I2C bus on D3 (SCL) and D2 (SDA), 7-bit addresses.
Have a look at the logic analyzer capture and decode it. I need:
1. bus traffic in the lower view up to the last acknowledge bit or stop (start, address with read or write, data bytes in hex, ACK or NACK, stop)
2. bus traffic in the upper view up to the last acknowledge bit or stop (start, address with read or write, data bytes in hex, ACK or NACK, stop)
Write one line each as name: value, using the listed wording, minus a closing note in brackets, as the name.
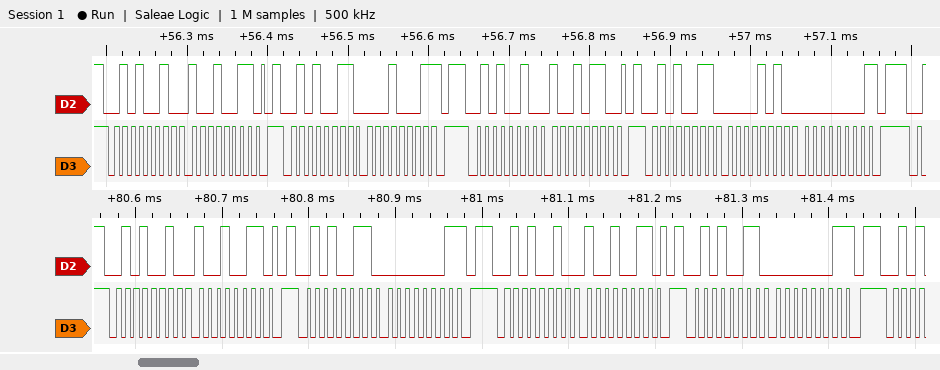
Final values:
bus traffic in the lower view up to the last acknowledge bit or stop: start, address 29 write ACK, 93 ACK, stop, start, address 29 read ACK, 01 NACK, stop, start, address 29 write ACK, 93 ACK, stop, start, address 29 read ACK, 01 NACK, stop
bus traffic in the upper view up to the last acknowledge bit or stop: start, address 29 write ACK, 93 ACK, stop, start, address 29 read ACK, 11 NACK, stop, start, address 29 write ACK, 96 ACK, stop, start, address 29 read ACK, 0A ACK, 00 NACK, stop
